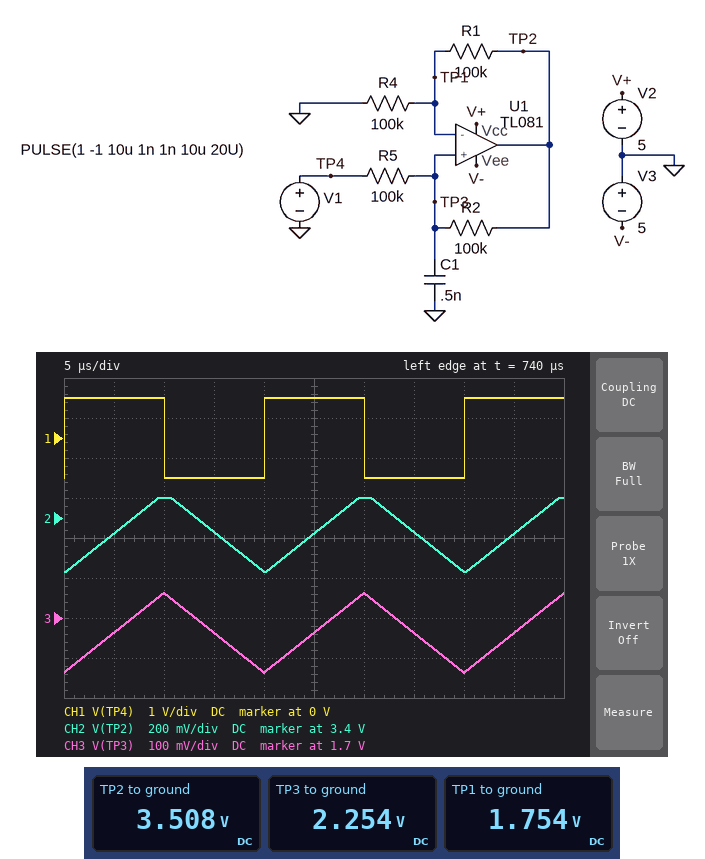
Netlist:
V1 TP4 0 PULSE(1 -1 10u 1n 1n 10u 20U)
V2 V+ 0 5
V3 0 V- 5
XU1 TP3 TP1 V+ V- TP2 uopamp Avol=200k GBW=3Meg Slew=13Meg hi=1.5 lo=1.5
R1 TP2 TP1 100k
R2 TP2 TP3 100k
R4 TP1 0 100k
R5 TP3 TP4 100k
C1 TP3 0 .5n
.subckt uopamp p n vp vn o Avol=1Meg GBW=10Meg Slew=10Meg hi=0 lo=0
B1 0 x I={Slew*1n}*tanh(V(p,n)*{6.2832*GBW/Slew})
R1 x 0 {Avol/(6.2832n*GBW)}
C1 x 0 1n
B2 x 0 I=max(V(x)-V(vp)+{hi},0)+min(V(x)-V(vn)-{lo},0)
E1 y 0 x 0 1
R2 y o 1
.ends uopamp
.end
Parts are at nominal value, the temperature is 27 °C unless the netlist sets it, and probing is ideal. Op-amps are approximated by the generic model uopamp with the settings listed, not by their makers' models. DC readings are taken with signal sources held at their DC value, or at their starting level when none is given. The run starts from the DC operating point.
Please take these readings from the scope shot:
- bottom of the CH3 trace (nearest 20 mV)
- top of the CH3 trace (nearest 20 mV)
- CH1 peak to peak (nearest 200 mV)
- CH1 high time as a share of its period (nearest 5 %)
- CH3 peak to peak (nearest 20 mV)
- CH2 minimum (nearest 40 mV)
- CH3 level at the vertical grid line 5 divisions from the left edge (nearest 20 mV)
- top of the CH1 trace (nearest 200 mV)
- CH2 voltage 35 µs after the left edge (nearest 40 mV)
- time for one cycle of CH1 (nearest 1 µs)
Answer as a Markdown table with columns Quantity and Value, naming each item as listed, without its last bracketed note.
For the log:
| Quantity | Value |
|---|---|
| bottom of the CH3 trace | 1.56 V |
| top of the CH3 trace | 1.76 V |
| CH1 peak to peak | 2.0 V |
| CH1 high time as a share of its period | 50 % |
| CH3 peak to peak | 200 mV |
| CH2 minimum | 3.12 V |
| CH3 level at the vertical grid line 5 divisions from the left edge | 1.66 V |
| top of the CH1 trace | 1.0 V |
| CH2 voltage 35 µs after the left edge | 3.32 V |
| time for one cycle of CH1 | 20 µs |
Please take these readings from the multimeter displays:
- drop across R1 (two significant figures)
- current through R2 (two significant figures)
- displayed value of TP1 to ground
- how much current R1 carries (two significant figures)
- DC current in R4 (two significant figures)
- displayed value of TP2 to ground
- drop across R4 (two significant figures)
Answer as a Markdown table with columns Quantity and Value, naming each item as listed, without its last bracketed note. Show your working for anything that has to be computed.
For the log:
| Quantity | Value |
|---|---|
| drop across R1 | 3.508 V - 1.754 V = 1.8 V |
| current through R2 | (3.508 V - 2.254 V) / 100 kΩ = 13 µA |
| displayed value of TP1 to ground | 1.754 V |
| how much current R1 carries | (3.508 V - 1.754 V) / 100 kΩ = 18 µA |
| DC current in R4 | (1.754 V) / 100 kΩ = 18 µA |
| displayed value of TP2 to ground | 3.508 V |
| drop across R4 | 1.754 V = 1.8 V |
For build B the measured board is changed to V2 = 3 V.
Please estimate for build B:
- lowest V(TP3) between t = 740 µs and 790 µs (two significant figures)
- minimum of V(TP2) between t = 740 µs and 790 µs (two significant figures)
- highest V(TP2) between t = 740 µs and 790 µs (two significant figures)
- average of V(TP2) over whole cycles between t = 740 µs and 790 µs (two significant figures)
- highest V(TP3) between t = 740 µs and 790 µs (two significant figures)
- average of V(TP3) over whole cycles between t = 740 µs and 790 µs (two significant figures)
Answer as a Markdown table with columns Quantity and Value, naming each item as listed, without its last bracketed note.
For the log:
| Quantity | Value |
|---|---|
| lowest V(TP3) between t = 740 µs and 790 µs | 560 mV |
| minimum of V(TP2) between t = 740 µs and 790 µs | 1.1 V |
| highest V(TP2) between t = 740 µs and 790 µs | 1.5 V |
| average of V(TP2) over whole cycles between t = 740 µs and 790 µs | 1.3 V |
| highest V(TP3) between t = 740 µs and 790 µs | 760 mV |
| average of V(TP3) over whole cycles between t = 740 µs and 790 µs | 660 mV |
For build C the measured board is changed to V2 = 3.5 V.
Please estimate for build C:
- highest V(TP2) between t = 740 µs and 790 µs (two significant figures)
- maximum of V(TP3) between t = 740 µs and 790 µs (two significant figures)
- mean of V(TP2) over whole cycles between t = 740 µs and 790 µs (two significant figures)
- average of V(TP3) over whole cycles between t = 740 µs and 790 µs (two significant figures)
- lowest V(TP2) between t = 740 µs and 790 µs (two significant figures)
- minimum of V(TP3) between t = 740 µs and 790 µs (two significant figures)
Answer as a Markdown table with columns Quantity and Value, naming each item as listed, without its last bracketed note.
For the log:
| Quantity | Value |
|---|---|
| highest V(TP2) between t = 740 µs and 790 µs | 2.0 V |
| maximum of V(TP3) between t = 740 µs and 790 µs | 1.0 V |
| mean of V(TP2) over whole cycles between t = 740 µs and 790 µs | 1.8 V |
| average of V(TP3) over whole cycles between t = 740 µs and 790 µs | 910 mV |
| lowest V(TP2) between t = 740 µs and 790 µs | 1.6 V |
| minimum of V(TP3) between t = 740 µs and 790 µs | 810 mV |
